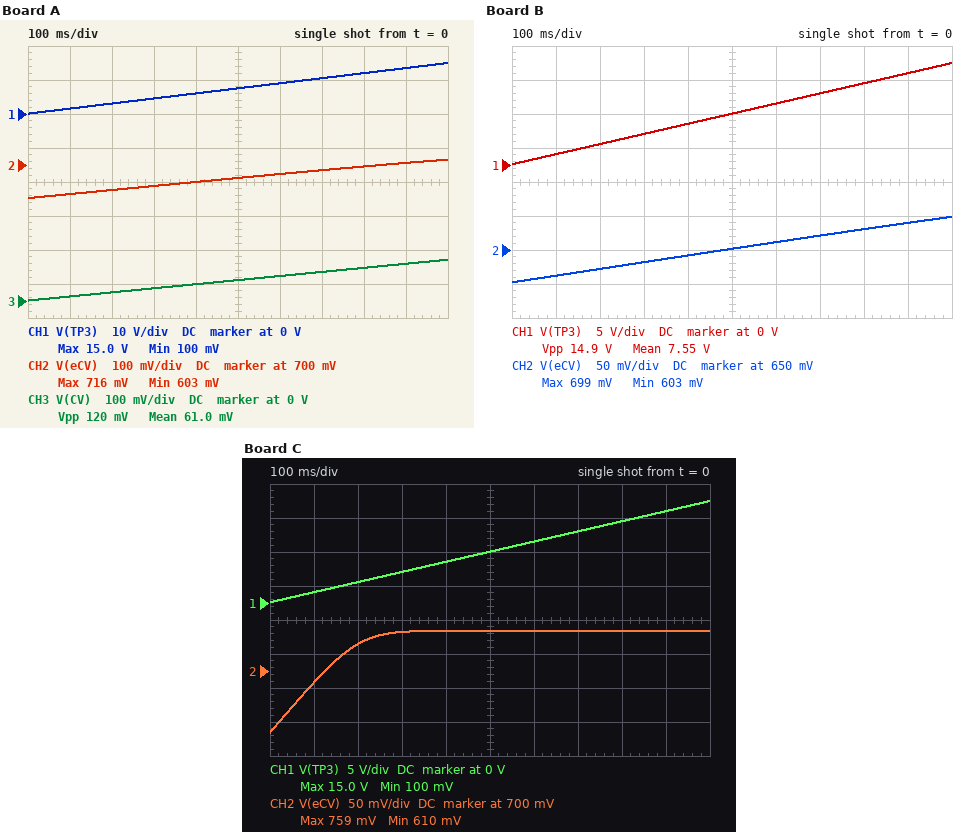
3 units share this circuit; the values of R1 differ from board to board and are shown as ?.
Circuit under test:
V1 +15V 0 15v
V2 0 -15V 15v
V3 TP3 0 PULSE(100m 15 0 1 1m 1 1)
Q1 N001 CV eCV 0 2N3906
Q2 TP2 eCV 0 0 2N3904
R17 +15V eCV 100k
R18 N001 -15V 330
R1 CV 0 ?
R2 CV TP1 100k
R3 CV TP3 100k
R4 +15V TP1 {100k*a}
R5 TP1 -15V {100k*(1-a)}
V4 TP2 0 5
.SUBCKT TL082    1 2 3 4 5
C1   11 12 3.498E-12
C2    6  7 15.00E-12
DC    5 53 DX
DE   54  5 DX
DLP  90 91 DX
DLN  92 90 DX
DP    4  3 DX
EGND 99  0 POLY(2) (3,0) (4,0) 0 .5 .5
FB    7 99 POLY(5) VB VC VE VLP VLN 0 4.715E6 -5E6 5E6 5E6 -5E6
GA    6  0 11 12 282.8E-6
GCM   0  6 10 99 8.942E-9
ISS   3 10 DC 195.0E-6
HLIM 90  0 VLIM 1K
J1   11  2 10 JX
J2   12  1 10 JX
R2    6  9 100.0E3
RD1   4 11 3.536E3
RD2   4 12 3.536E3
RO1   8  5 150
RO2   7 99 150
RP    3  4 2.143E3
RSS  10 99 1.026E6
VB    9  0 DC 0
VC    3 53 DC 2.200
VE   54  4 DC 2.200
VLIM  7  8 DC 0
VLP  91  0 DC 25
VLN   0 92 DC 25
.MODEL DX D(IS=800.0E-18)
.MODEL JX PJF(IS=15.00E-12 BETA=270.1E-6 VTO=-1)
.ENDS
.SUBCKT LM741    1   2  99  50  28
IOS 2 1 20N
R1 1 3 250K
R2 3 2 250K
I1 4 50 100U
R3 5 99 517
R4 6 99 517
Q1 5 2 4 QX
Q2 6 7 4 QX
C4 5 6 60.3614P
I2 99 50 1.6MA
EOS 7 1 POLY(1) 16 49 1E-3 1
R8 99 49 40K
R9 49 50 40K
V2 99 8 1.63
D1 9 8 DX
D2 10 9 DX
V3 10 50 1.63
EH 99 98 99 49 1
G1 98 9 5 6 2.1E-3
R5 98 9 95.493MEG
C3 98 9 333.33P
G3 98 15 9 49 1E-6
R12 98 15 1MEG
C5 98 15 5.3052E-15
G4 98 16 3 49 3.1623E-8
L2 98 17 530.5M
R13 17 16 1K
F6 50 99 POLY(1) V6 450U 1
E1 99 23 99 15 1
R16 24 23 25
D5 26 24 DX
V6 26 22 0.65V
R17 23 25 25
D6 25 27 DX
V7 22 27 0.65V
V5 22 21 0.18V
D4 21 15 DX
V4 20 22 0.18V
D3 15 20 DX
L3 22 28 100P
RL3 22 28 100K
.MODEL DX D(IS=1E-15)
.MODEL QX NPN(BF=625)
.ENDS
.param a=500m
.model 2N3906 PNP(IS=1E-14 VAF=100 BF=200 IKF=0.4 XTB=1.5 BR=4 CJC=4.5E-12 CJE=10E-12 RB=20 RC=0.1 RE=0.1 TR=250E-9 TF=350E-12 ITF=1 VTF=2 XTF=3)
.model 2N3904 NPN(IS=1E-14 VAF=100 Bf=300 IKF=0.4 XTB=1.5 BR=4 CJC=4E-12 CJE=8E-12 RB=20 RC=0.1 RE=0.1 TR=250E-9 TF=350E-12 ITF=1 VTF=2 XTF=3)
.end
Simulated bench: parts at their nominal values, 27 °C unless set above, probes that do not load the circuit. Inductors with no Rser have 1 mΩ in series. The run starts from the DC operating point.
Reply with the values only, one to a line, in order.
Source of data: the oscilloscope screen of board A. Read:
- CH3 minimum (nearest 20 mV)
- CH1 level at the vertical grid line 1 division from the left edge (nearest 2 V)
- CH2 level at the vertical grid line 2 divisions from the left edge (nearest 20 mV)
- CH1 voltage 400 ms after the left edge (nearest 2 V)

0 V
2 V
620 mV
6 V
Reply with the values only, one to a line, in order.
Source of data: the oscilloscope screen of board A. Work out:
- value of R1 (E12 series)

820 Ω
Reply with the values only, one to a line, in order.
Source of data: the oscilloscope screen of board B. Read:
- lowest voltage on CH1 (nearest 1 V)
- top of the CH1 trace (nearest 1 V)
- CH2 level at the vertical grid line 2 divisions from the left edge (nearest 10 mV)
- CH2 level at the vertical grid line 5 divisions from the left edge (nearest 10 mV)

0 V
15 V
620 mV
650 mV
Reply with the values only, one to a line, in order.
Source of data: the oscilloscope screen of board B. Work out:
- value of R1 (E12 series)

680 Ω
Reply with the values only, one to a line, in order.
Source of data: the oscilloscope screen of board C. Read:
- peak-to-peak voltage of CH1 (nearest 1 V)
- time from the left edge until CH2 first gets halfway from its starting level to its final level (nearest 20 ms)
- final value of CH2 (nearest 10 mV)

15 V
100 ms
760 mV
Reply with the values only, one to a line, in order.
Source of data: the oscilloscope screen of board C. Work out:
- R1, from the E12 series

5.6 kΩ
